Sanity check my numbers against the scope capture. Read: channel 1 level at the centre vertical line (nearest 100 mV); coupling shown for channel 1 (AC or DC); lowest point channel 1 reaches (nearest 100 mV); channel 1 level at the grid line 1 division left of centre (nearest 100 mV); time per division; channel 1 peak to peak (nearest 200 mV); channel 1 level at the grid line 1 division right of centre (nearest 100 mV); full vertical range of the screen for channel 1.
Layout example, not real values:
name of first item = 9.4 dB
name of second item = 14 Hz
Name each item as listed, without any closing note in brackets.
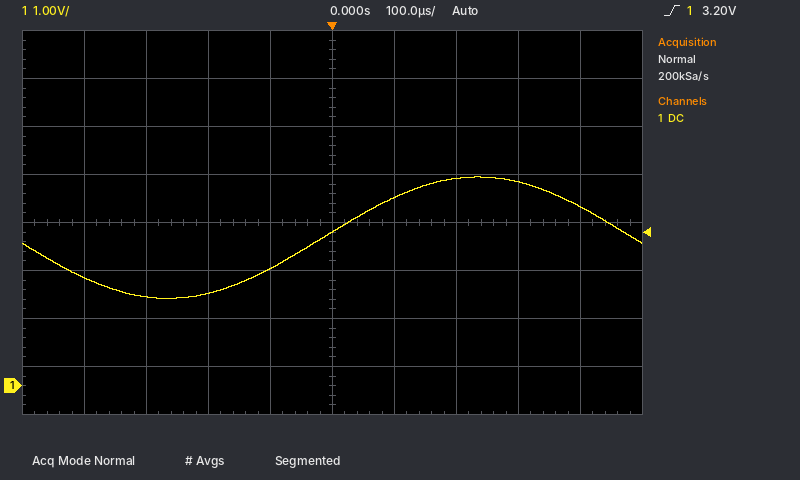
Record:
channel 1 level at the centre vertical line = 3.2 V
coupling shown for channel 1 = DC
lowest point channel 1 reaches = 1.8 V
channel 1 level at the grid line 1 division left of centre = 2.4 V
time per division = 100 µs
channel 1 peak to peak = 2.6 V
channel 1 level at the grid line 1 division right of centre = 3.9 V
full vertical range of the screen for channel 1 = 8 V
